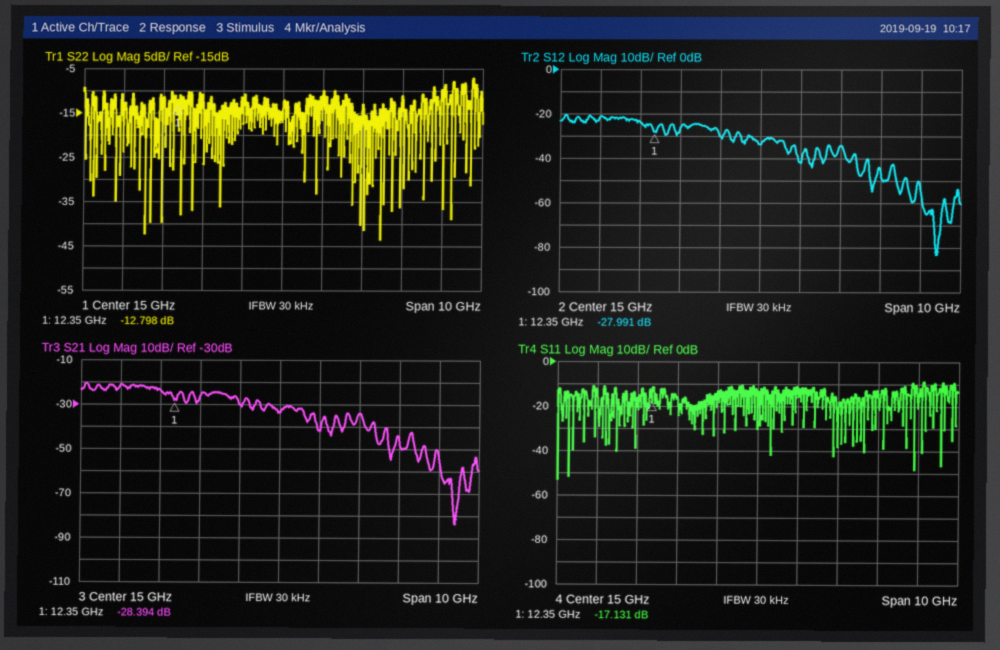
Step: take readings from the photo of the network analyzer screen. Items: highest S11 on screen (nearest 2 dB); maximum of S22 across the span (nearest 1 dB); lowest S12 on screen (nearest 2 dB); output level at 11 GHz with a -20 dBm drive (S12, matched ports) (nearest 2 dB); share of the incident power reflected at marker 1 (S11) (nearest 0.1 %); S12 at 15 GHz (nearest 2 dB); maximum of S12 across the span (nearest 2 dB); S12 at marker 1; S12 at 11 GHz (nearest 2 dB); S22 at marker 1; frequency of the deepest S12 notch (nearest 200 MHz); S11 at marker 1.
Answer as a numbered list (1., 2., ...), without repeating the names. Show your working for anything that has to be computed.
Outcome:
1. -8 dB
2. -7 dB
3. -84 dB
4. -20 dBm + (-22 dB) = -42 dBm
5. 10^(-17.131/10) ≈ 1.9 %
6. -34 dB
7. -20 dB
8. -27.991 dB
9. -22 dB
10. -12.798 dB
11. 19.4 GHz
12. -17.131 dB
